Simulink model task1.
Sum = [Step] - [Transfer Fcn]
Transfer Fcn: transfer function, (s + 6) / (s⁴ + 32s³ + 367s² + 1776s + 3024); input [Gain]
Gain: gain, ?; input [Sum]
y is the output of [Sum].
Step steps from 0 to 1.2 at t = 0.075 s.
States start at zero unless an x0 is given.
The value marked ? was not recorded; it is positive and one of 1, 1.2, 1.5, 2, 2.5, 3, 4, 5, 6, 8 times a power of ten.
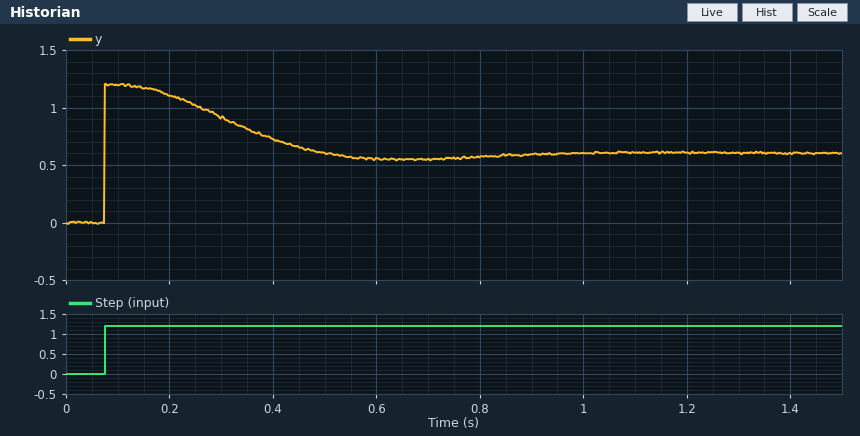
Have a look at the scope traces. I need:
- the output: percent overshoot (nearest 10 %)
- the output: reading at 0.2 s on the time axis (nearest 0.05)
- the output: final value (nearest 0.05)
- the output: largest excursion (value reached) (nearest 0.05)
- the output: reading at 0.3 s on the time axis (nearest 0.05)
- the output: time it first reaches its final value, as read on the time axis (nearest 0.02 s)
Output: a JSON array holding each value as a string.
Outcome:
["100 %", "1.10", "0.60", "1.20", "0.90", "0.08 s"]
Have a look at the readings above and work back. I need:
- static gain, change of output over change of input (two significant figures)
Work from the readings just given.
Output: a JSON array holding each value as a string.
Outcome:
["0.50"]
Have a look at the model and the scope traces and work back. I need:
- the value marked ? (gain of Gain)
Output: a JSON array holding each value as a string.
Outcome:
["500"]
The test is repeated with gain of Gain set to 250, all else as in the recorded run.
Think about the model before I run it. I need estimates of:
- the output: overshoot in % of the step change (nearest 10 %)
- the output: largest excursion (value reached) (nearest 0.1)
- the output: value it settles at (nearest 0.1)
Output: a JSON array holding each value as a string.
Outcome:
["50 %", "1.2", "0.8"]
